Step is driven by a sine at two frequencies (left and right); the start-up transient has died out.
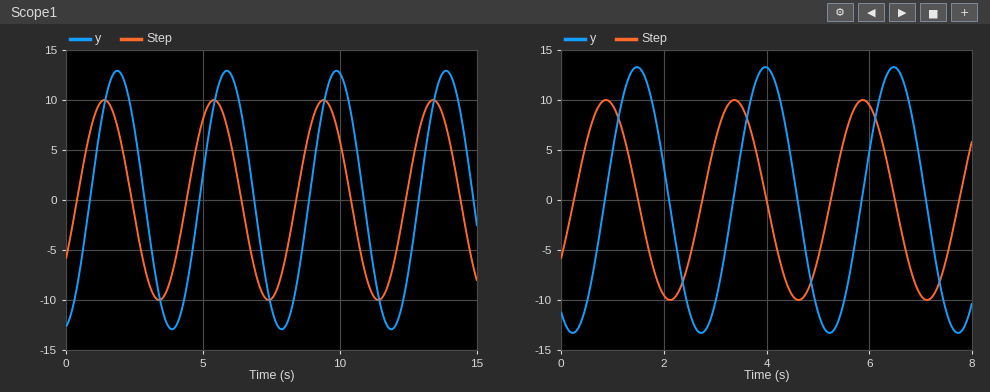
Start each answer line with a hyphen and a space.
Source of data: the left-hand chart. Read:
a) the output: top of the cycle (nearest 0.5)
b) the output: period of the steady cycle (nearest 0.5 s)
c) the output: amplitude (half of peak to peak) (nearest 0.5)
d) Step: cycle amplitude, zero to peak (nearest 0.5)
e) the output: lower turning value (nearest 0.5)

- 13.0
- 4.0 s
- 13.0
- 10.0
- -13.0
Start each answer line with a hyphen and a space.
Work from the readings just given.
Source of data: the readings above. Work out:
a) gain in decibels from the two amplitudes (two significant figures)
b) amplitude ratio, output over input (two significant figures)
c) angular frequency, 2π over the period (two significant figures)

- 2.3 dB
- 1.3
- 1.6 rad/s
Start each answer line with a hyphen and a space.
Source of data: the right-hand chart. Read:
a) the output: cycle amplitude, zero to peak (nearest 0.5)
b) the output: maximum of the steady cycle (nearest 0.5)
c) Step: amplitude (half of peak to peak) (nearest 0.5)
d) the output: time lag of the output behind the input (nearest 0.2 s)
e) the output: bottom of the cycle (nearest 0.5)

- 13.5
- 13.5
- 10.0
- 0.6 s
- -13.5
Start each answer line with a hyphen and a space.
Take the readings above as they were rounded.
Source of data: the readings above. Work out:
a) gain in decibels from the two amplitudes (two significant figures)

- 2.6 dB
